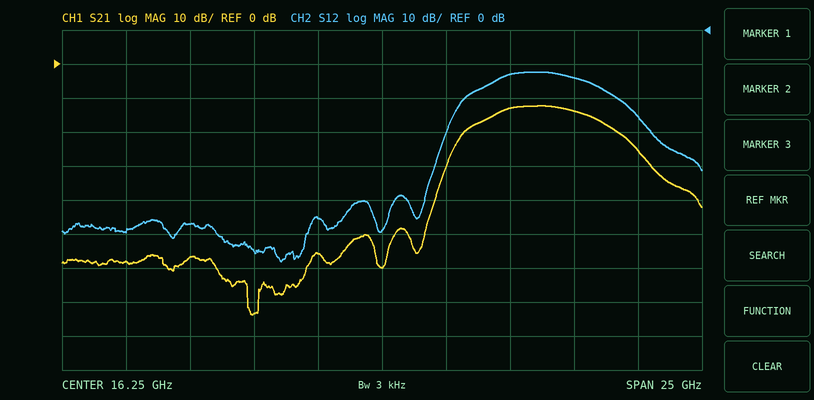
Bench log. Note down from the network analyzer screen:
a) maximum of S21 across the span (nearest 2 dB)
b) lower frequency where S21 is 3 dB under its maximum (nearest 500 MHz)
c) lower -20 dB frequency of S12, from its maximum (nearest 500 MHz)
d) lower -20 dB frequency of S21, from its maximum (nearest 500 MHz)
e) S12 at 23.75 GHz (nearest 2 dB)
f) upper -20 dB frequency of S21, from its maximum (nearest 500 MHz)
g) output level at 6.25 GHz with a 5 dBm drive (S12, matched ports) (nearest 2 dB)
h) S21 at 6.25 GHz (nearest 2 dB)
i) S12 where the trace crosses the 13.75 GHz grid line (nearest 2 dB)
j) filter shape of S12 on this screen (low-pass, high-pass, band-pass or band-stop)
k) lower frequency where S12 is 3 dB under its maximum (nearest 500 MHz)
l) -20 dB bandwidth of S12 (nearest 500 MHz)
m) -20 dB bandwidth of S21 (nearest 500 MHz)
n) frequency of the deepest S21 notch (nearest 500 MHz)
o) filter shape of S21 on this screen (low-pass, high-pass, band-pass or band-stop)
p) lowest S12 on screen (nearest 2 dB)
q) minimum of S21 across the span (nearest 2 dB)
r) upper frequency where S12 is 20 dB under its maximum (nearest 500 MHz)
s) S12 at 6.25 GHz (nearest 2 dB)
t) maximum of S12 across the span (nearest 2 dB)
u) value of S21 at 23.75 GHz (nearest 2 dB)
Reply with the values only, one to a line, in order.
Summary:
-12 dB
20.5 GHz
18.5 GHz
18.5 GHz
-14 dB
27.0 GHz
-54 dBm
-58 dB
-56 dB
band-pass
20.5 GHz
8.5 GHz
8.5 GHz
11.0 GHz
band-pass
-68 dB
-74 dB
27.0 GHz
-60 dB
-12 dB
-14 dB
